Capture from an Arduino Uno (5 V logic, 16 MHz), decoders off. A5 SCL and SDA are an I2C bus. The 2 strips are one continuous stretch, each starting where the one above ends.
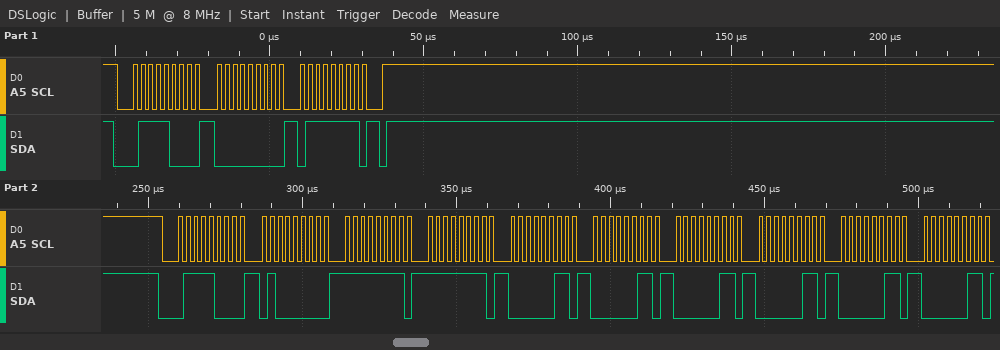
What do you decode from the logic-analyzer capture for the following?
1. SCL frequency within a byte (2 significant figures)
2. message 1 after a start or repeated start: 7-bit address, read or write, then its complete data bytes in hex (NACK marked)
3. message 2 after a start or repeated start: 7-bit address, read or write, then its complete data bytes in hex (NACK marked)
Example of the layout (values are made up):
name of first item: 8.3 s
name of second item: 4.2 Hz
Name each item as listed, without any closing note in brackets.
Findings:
SCL frequency within a byte: 400 kHz
message 1 after a start or repeated start: 7-bit address, read or write, then its complete data bytes in hex: 0x3C write: 00 7F
message 2 after a start or repeated start: 7-bit address, read or write, then its complete data bytes in hex: 0x3C write: 40 FF FF 03 03 03 03 03 03
